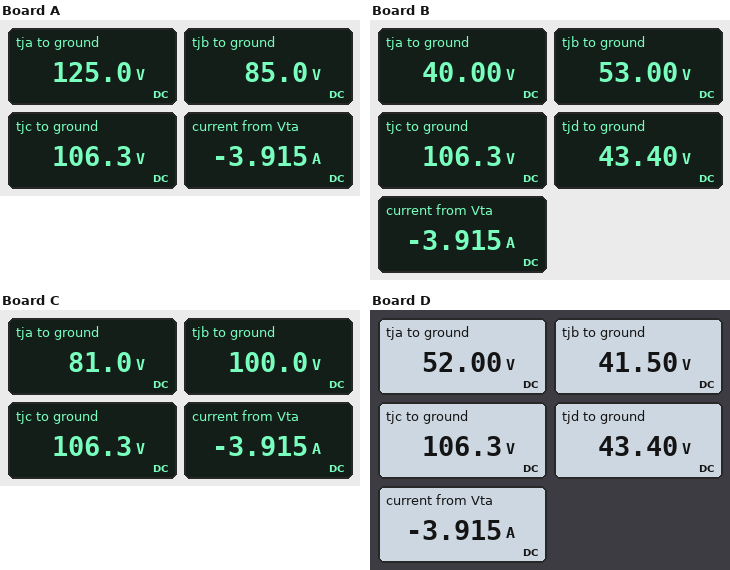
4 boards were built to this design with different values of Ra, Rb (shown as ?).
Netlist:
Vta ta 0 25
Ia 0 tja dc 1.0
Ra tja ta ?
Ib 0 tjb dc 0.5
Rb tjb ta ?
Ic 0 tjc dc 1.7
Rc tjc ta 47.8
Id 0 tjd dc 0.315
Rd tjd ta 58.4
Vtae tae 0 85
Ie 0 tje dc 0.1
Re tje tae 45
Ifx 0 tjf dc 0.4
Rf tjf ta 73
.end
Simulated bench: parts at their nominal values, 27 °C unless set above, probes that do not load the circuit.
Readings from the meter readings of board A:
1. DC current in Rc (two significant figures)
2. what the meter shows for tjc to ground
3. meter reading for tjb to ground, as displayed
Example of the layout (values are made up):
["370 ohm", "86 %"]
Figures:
["1.7 A", "106.3 V", "85.0 V"]
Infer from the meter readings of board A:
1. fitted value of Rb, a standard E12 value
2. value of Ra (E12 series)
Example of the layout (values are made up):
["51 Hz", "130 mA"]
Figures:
["120 Ω", "100 Ω"]
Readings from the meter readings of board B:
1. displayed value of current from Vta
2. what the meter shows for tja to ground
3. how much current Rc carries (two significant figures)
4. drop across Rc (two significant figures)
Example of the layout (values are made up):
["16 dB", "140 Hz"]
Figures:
["-3.915 A", "40.00 V", "1.7 A", "81 V"]
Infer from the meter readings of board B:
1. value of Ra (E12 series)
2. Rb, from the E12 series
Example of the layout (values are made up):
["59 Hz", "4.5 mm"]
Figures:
["15 Ω", "56 Ω"]
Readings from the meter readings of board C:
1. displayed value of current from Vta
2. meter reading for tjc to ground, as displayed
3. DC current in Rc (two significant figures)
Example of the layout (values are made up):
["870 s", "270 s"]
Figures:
["-3.915 A", "106.3 V", "1.7 A"]
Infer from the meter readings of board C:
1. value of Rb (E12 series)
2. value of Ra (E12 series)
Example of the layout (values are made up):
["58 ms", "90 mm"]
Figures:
["150 Ω", "56 Ω"]
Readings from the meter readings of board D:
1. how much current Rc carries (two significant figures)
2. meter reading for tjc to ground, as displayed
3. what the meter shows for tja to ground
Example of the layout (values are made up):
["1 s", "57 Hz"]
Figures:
["1.7 A", "106.3 V", "52.00 V"]
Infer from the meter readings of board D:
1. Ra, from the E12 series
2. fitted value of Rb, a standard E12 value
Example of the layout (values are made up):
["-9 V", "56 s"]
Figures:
["27 Ω", "33 Ω"]
